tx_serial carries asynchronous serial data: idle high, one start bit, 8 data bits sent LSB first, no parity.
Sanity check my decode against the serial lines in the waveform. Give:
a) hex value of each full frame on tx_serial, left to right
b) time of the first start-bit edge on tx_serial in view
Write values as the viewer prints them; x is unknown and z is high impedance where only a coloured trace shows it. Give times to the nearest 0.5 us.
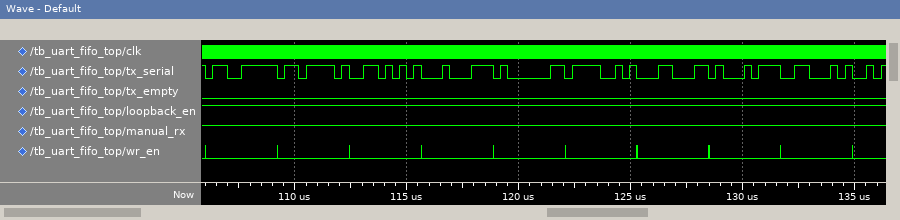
F3, 7B, 56, C4, 81, 4F, 8C, D1, 46
106 us
